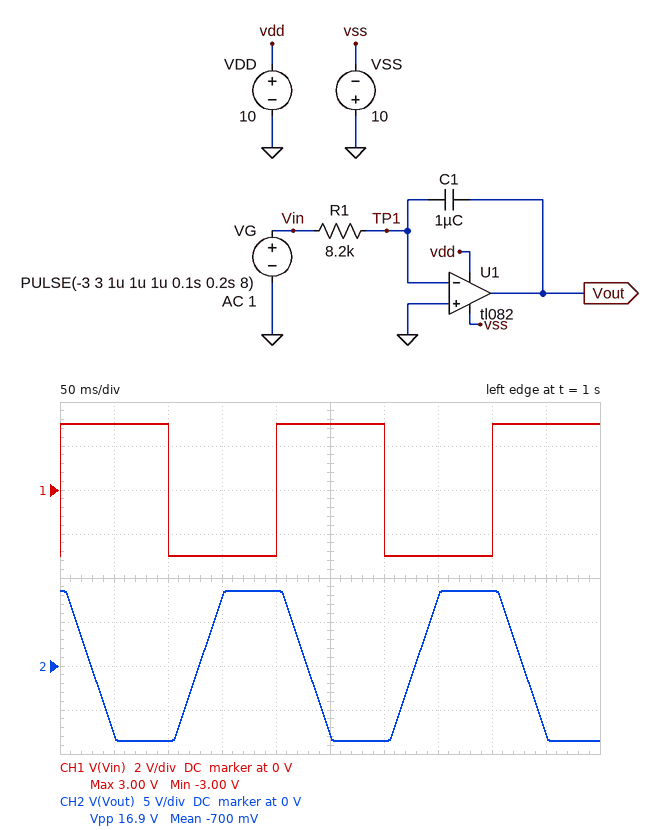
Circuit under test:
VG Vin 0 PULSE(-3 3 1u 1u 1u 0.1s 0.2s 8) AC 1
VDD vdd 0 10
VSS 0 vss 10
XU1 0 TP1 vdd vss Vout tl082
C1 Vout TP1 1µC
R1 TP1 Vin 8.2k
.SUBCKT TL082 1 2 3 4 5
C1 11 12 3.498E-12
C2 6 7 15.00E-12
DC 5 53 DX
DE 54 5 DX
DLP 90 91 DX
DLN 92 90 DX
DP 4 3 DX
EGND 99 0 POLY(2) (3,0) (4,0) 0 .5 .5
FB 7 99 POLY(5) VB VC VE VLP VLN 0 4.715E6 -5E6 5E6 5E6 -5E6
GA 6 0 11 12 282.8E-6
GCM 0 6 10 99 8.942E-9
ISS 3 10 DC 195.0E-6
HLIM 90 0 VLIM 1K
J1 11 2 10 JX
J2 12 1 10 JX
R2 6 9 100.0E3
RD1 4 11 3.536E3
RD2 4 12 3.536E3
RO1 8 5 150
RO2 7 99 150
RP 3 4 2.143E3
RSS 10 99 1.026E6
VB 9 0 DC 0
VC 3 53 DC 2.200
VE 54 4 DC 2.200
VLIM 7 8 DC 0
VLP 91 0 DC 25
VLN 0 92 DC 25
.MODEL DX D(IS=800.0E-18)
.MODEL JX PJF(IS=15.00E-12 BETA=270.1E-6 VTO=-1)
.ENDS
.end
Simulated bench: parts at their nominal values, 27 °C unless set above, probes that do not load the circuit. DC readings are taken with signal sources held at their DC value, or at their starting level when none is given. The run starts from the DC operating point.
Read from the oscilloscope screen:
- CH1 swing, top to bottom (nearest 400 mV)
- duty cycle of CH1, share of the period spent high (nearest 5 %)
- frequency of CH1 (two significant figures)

6.0 V
50 %
5.0 Hz
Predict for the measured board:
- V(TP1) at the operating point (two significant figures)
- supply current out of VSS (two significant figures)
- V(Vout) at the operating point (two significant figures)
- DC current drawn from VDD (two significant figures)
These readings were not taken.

-3.0 V
9.5 mA
8.5 V
9.3 mA
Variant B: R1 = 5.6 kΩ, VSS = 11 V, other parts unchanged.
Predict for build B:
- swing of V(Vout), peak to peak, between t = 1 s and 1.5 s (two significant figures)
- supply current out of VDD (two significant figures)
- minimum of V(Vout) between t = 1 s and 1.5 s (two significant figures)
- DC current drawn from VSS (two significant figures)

18 V
9.8 mA
-9.5 V
10 mA
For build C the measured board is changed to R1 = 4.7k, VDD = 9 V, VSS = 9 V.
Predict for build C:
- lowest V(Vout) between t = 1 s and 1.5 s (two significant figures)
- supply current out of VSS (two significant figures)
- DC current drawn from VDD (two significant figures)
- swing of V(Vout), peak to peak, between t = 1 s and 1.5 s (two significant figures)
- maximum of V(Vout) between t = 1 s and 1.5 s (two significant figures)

-7.5 V
8.6 mA
8.4 mA
15 V
7.5 V
